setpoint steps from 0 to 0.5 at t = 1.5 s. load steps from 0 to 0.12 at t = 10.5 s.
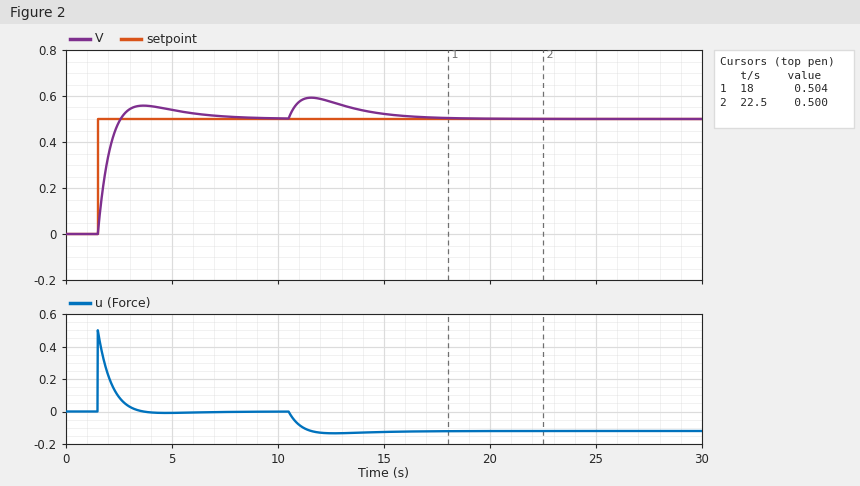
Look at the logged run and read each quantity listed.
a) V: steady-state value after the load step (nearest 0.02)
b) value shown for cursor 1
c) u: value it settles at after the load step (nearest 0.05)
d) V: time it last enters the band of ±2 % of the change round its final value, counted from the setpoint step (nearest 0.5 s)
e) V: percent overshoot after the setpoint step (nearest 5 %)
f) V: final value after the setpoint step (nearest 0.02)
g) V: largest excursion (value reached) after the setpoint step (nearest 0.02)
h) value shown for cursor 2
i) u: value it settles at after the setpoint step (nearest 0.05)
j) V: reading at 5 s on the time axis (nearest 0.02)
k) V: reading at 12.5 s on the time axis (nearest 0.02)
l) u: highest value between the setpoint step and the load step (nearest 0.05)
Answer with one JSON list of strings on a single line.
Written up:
["0.50", "0.504", "-0.10", "6.0 s", "10 %", "0.50", "0.56", "0.500", "0.00", "0.54", "0.58", "0.50"]
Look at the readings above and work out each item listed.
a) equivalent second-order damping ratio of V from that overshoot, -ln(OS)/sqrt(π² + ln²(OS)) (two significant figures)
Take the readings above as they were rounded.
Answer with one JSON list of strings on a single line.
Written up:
["0.59"]
